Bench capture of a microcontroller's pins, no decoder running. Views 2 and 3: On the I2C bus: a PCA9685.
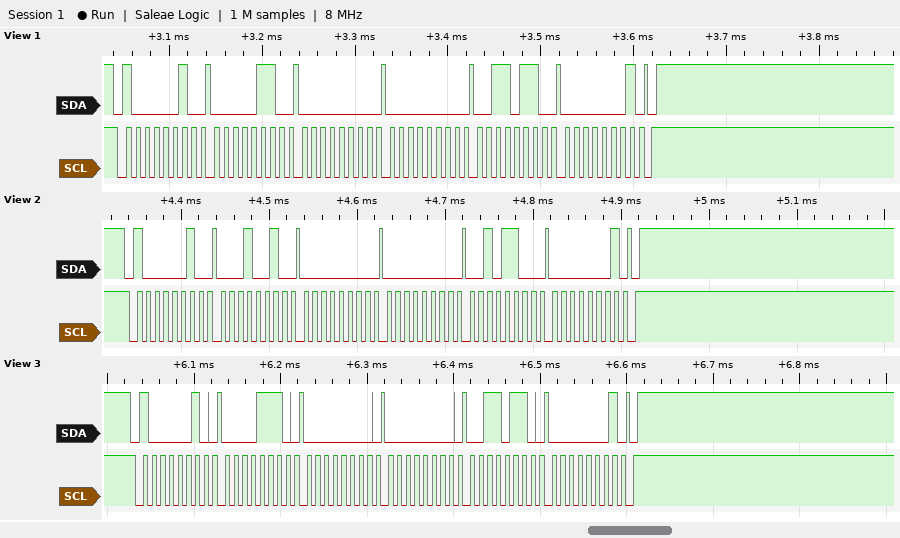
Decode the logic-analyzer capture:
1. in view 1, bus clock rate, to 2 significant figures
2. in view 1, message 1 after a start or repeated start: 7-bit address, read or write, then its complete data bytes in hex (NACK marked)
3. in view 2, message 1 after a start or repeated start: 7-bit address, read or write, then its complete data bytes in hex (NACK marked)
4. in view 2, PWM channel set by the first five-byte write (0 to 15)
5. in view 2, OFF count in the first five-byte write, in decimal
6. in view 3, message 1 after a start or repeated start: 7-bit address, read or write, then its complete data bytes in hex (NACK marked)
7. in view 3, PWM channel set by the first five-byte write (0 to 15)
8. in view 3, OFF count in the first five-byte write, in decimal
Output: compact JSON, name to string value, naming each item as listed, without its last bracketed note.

{"in view 1, bus clock rate, to 2 significant figures": "100 kHz", "in view 1, message 1 after a start or repeated start: 7-bit address, read or write, then its complete data bytes in hex": "0x41 write: 06 00 00 36 01", "in view 2, message 1 after a start or repeated start: 7-bit address, read or write, then its complete data bytes in hex": "0x41 write: 12 00 00 2C 01", "in view 2, PWM channel set by the first five-byte write": "3", "in view 2, OFF count in the first five-byte write, in decimal": "300", "in view 3, message 1 after a start or repeated start: 7-bit address, read or write, then its complete data bytes in hex": "0x41 write: 0E 00 00 36 01", "in view 3, PWM channel set by the first five-byte write": "2", "in view 3, OFF count in the first five-byte write, in decimal": "310"}
